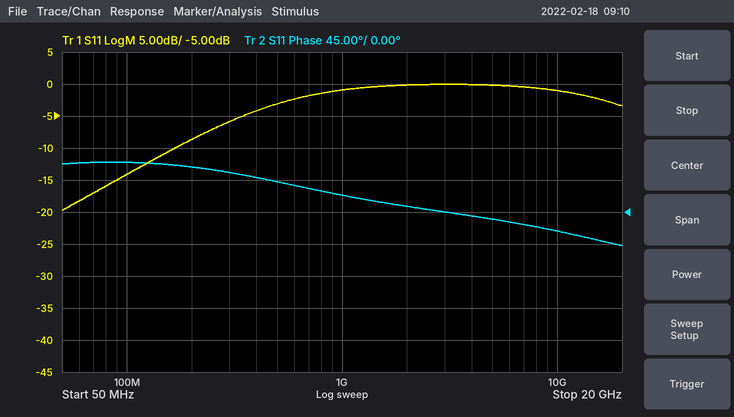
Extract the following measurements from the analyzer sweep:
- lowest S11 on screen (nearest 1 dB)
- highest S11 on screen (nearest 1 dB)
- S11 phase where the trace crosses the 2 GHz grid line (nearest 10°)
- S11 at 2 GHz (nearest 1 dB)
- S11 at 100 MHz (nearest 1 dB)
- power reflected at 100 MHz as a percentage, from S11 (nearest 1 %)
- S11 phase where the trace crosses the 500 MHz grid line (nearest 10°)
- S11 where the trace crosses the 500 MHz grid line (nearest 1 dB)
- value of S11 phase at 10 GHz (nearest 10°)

-20 dB
0 dB
10°
0 dB
-14 dB
4 %
40°
-3 dB
-30°
